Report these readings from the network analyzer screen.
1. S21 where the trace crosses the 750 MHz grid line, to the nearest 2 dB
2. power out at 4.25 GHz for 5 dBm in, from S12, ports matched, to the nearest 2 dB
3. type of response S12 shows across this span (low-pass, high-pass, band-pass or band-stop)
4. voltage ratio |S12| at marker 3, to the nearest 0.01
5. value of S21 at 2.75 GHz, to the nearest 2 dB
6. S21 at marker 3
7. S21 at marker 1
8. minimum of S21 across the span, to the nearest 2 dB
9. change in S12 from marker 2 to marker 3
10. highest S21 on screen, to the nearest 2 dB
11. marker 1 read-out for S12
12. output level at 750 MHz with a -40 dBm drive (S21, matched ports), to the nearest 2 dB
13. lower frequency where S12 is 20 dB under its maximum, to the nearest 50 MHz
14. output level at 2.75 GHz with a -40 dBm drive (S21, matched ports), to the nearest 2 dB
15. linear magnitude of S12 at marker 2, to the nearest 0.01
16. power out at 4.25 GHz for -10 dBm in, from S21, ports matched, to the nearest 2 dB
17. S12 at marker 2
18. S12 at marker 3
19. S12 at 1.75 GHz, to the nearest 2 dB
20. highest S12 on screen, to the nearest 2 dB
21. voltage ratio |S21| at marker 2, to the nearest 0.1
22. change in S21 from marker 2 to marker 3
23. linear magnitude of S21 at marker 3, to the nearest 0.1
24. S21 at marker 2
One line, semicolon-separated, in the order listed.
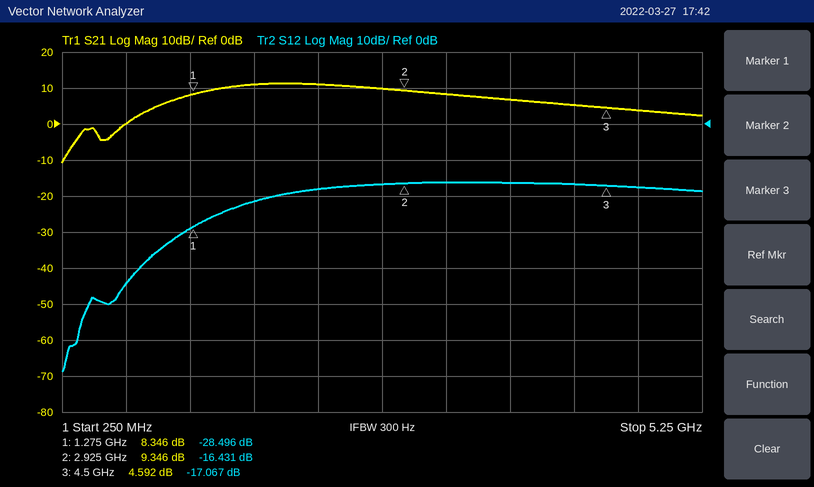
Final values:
0 dB; -12 dBm; high-pass; 0.14; 10 dB; 4.592 dB; 8.346 dB; -10 dB; -0.636 dB; 12 dB; -28.496 dB; -40 dBm; 950 MHz; -30 dBm; 0.15; -4 dBm; -16.431 dB; -17.067 dB; -22 dB; -16 dB; 2.9; -4.754 dB; 1.7; 9.346 dB
